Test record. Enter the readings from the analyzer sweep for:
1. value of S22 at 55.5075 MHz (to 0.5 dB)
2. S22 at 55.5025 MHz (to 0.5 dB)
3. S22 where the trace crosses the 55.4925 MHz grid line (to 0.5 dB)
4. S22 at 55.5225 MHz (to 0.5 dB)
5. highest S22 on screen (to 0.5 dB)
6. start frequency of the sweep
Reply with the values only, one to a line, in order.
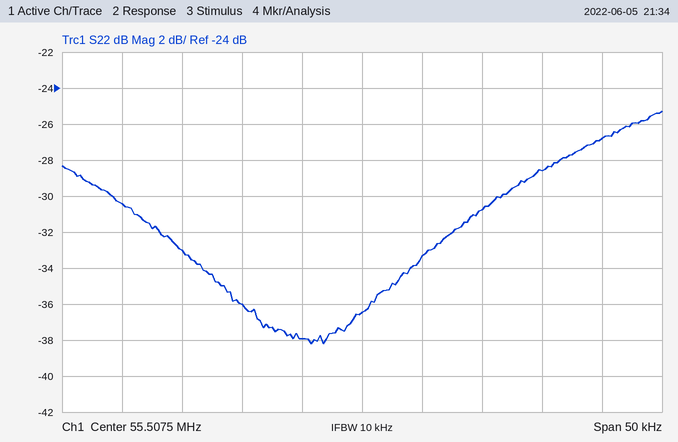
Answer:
-36.5 dB
-38.0 dB
-33.0 dB
-28.5 dB
-25.5 dB
55.4825 MHz
